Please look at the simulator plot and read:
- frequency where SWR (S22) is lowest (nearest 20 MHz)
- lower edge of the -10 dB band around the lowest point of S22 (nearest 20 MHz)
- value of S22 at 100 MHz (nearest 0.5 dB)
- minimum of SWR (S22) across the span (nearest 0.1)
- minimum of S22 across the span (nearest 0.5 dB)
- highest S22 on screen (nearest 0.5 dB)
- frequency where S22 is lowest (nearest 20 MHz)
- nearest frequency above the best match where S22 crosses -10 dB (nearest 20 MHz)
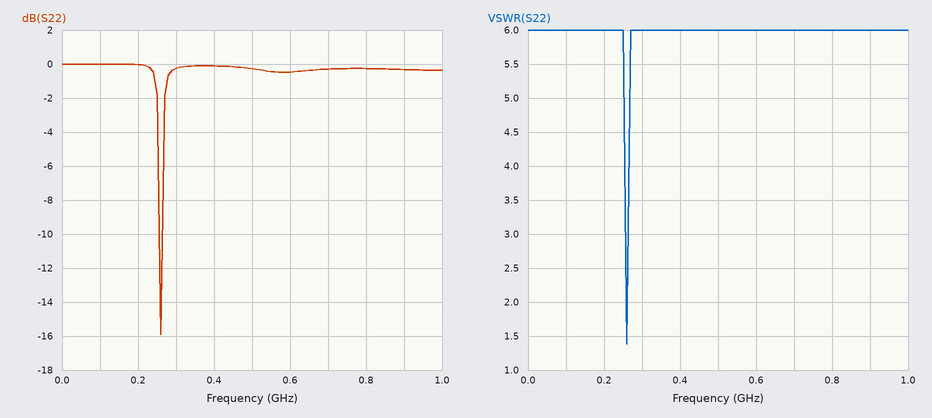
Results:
260 MHz
260 MHz
0.0 dB
1.4
-16.0 dB
0.0 dB
260 MHz
260 MHz
